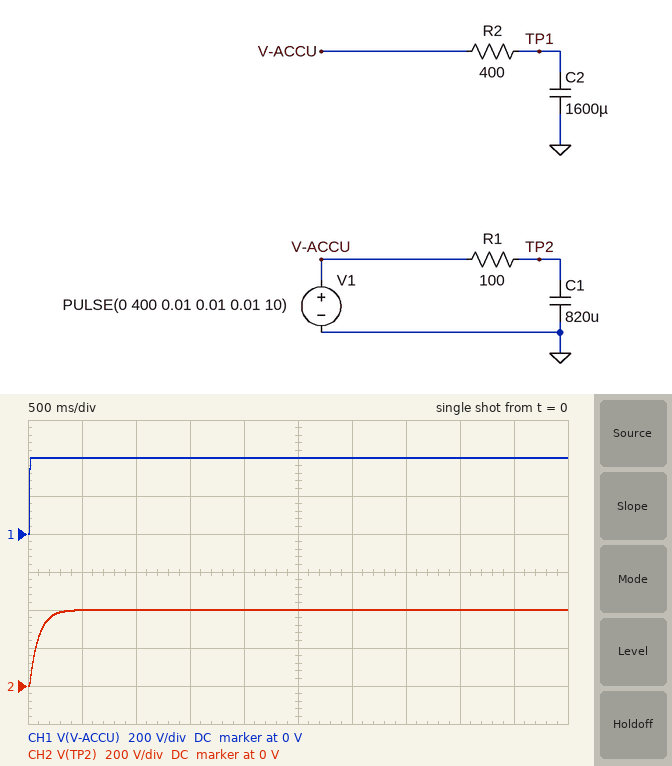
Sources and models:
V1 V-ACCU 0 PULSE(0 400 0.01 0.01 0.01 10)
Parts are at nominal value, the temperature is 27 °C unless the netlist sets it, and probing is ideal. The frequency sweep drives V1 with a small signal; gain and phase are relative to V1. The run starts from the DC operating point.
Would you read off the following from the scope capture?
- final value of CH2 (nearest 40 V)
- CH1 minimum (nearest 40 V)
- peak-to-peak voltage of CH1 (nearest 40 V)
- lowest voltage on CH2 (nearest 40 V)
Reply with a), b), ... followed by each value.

a) 400 V
b) 0 V
c) 400 V
d) 0 V
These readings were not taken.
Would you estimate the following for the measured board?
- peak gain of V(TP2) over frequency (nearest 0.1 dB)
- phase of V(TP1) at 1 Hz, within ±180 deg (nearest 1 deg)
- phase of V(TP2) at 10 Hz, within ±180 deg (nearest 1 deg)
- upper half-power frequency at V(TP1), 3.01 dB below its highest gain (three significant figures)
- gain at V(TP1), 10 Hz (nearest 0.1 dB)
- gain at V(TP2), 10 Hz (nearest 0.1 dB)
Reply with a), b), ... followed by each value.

a) 0 dB
b) -76 deg
c) -79 deg
d) 249 mHz
e) -32.1 dB
f) -14.4 dB
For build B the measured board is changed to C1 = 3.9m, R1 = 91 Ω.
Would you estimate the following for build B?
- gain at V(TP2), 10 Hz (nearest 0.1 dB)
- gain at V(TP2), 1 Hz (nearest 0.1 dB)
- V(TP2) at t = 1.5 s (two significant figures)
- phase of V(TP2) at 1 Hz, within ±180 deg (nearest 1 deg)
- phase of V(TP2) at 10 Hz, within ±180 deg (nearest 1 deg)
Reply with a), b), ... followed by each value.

a) -27.0 dB
b) -7.8 dB
c) 390 V
d) -66 deg
e) -87 deg
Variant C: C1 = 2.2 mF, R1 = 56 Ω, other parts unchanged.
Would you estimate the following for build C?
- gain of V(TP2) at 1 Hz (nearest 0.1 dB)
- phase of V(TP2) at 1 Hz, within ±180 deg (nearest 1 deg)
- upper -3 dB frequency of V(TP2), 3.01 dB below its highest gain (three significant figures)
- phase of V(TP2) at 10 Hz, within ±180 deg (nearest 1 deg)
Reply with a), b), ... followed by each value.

a) -2.0 dB
b) -38 deg
c) 1.29 Hz
d) -83 deg
